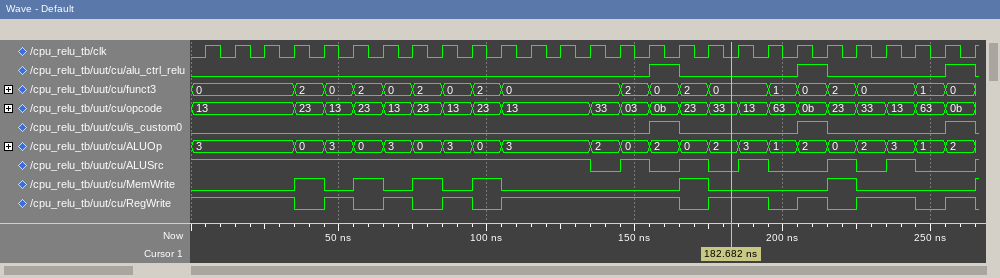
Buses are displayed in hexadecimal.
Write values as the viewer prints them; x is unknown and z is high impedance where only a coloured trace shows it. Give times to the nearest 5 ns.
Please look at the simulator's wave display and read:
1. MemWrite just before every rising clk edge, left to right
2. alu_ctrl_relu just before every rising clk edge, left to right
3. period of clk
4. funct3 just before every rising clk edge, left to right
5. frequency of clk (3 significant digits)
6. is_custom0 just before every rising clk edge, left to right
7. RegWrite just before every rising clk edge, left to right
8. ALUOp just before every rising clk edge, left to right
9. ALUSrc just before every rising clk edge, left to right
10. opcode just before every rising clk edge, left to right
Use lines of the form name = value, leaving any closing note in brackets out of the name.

MemWrite just before every rising clk edge, left to right = 0 0 0 0 1 0 1 0 1 0 1 0 0 0 0 0 0 1 0 0 0 0 1 0 0 0 0
alu_ctrl_relu just before every rising clk edge, left to right = 0 0 0 0 0 0 0 0 0 0 0 0 0 0 0 0 1 0 0 0 0 1 0 0 0 0 1
period of clk = 10 ns
funct3 just before every rising clk edge, left to right = 0, 0, 0, 0, 2, 0, 2, 0, 2, 0, 2, 0, 0, 0, 0, 2, 0, 2, 0, 0, 1, 0, 2, 0, 0, 1, 0
frequency of clk = 100 MHz
is_custom0 just before every rising clk edge, left to right = 0 0 0 0 0 0 0 0 0 0 0 0 0 0 0 0 1 0 0 0 0 1 0 0 0 0 1
RegWrite just before every rising clk edge, left to right = 1 1 1 1 0 1 0 1 0 1 0 1 1 1 1 1 1 0 1 1 0 1 0 1 1 0 1
ALUOp just before every rising clk edge, left to right = 3, 3, 3, 3, 0, 3, 0, 3, 0, 3, 0, 3, 3, 3, 2, 0, 2, 0, 2, 3, 1, 2, 0, 2, 3, 1, 2
ALUSrc just before every rising clk edge, left to right = 1 1 1 1 1 1 1 1 1 1 1 1 1 1 0 1 0 1 0 1 0 0 1 0 1 0 0
opcode just before every rising clk edge, left to right = 13, 13, 13, 13, 23, 13, 23, 13, 23, 13, 23, 13, 13, 13, 33, 03, 0b, 23, 33, 13, 63, 0b, 23, 33, 13, 63, 0b
